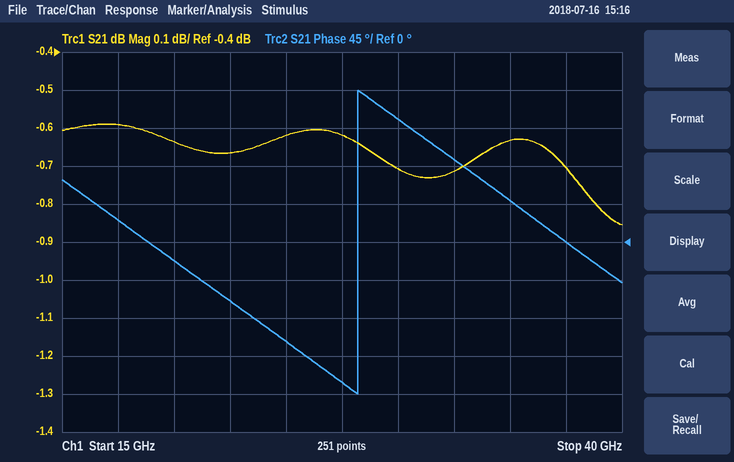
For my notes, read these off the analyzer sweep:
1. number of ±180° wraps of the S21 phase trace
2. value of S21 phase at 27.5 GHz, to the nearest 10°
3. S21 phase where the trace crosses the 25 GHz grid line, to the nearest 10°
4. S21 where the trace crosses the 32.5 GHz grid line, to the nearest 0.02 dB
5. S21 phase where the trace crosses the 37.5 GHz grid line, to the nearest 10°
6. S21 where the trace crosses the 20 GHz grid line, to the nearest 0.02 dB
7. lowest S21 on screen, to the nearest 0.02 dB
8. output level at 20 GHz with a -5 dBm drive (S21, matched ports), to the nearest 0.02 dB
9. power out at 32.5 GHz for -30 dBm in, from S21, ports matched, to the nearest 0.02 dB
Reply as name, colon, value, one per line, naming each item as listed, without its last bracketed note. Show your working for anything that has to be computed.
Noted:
number of ±180° wraps of the S21 phase trace: 1
value of S21 phase at 27.5 GHz, to the nearest 10°: -170°
S21 phase where the trace crosses the 25 GHz grid line, to the nearest 10°: -120°
S21 where the trace crosses the 32.5 GHz grid line, to the nearest 0.02 dB: -0.72 dB
S21 phase where the trace crosses the 37.5 GHz grid line, to the nearest 10°: 0°
S21 where the trace crosses the 20 GHz grid line, to the nearest 0.02 dB: -0.64 dB
lowest S21 on screen, to the nearest 0.02 dB: -0.86 dB
output level at 20 GHz with a -5 dBm drive (S21, matched ports), to the nearest 0.02 dB: -5 dBm + (-0.64 dB) = -5.64 dBm
power out at 32.5 GHz for -30 dBm in, from S21, ports matched, to the nearest 0.02 dB: -30 dBm + (-0.72 dB) = -30.72 dBm
